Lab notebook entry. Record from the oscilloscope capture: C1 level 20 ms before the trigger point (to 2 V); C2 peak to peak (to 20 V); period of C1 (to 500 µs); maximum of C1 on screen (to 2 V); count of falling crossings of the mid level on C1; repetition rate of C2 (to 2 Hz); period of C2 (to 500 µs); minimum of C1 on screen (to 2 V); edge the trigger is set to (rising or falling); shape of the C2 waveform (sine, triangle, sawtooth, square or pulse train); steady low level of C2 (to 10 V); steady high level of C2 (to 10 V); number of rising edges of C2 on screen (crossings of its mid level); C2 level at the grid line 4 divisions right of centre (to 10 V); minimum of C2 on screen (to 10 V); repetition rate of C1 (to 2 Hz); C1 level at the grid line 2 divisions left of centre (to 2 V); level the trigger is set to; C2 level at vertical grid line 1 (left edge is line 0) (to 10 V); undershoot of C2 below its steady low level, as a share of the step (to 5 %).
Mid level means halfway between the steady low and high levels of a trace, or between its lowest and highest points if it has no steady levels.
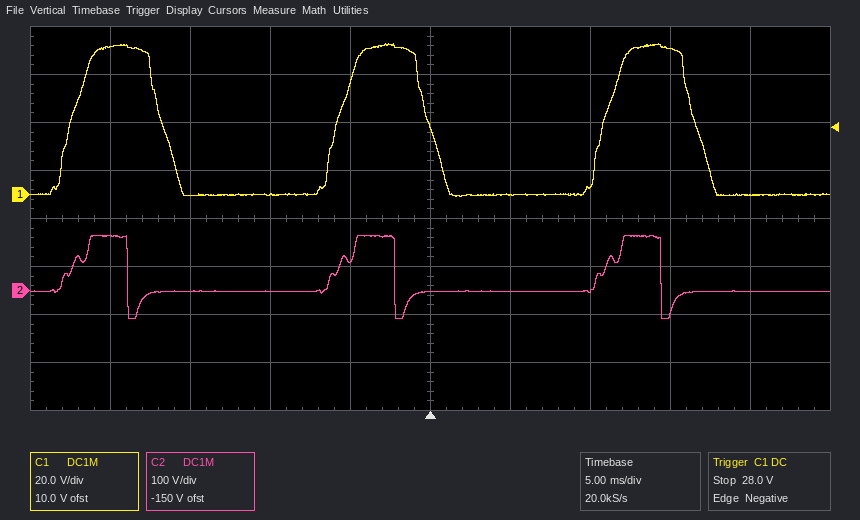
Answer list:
62 V
180 V
16.5 ms
62 V
3
60 Hz
16.5 ms
0 V
falling
pulse train
0 V
110 V
3
0 V
-60 V
60 Hz
0 V
28.0 V
110 V
50 %
